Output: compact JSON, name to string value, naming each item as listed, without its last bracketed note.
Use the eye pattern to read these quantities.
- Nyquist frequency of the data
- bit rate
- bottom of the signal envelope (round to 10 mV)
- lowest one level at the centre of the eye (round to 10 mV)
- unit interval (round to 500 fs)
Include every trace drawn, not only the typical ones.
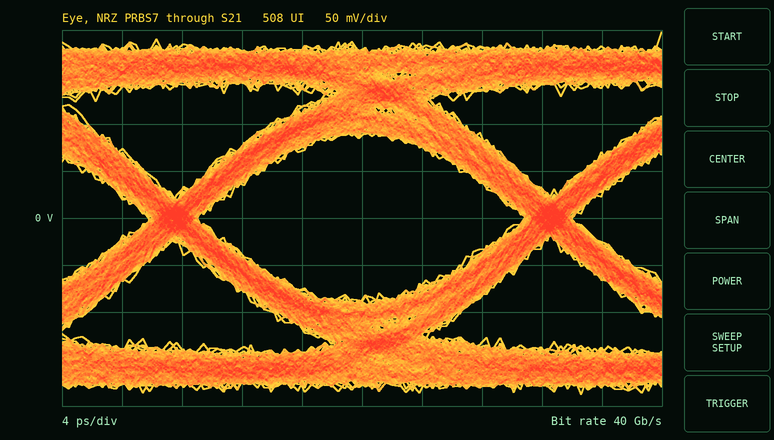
{"Nyquist frequency of the data": "20 GHz", "bit rate": "40 Gb/s", "bottom of the signal envelope": "-190 mV", "lowest one level at the centre of the eye": "90 mV", "unit interval": "25.0 ps"}
